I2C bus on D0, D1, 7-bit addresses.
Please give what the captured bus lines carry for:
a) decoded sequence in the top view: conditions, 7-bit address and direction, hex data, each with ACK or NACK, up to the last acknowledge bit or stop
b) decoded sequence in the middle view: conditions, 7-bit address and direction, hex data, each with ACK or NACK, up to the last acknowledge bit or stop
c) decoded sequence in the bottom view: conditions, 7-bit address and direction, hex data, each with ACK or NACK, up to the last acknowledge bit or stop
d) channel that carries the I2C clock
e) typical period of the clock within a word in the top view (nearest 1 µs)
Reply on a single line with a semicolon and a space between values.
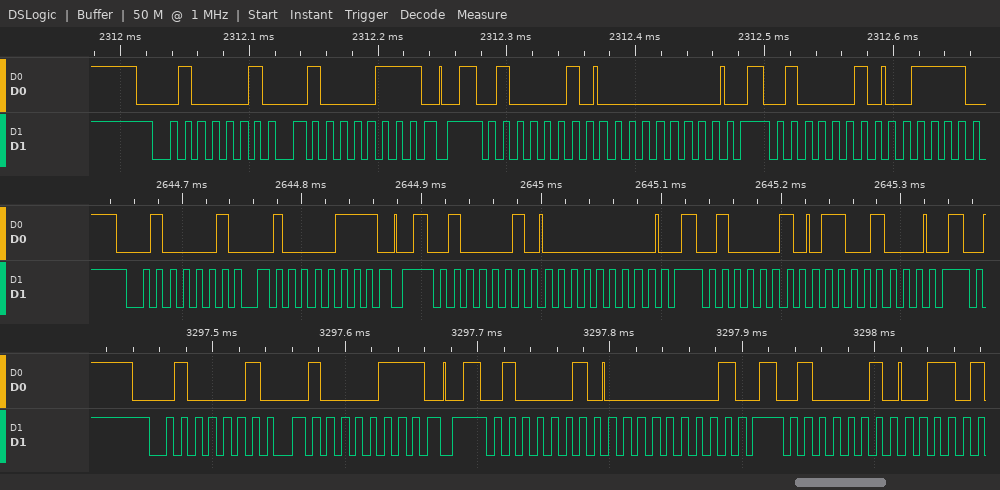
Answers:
start, address 21 write ACK, 87 ACK, stop, start, address 21 write ACK, 00 ACK, stop, start, address 21 write ACK; start, address 21 write ACK, 87 ACK, stop, start, address 21 write ACK, 00 ACK, stop, start, address 21 write ACK, C8 ACK, stop; start, address 21 write ACK, 87 ACK, stop, start, address 21 write ACK, 01 ACK, stop, start, address 21 write ACK; D1; 11 µs
